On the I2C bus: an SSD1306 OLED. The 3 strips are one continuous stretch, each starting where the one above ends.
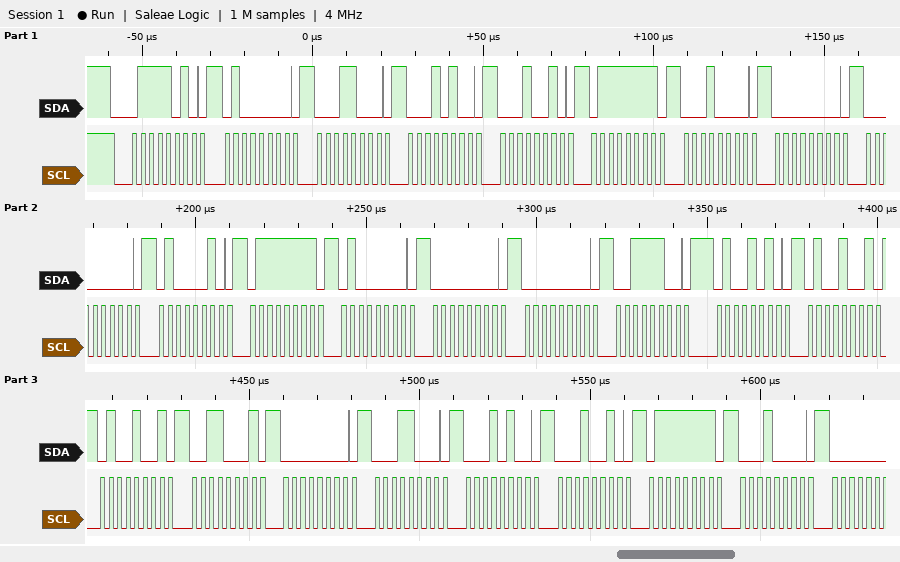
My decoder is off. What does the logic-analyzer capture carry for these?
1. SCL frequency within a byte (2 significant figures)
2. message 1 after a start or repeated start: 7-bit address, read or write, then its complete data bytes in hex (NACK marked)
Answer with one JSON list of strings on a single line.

["400 kHz", "0x3D write: 40 18 14 12 7F 10 00 00 42 7F 40 00 00 3C 4A 49 49 31 00 18 14 12 7F 10"]
